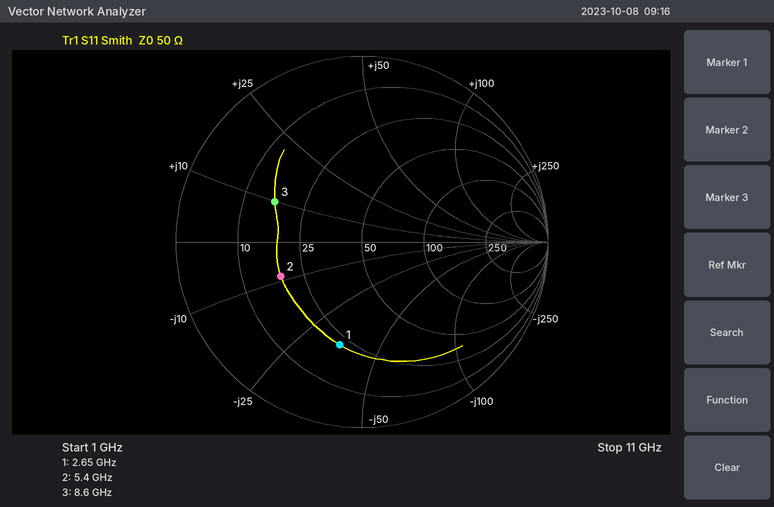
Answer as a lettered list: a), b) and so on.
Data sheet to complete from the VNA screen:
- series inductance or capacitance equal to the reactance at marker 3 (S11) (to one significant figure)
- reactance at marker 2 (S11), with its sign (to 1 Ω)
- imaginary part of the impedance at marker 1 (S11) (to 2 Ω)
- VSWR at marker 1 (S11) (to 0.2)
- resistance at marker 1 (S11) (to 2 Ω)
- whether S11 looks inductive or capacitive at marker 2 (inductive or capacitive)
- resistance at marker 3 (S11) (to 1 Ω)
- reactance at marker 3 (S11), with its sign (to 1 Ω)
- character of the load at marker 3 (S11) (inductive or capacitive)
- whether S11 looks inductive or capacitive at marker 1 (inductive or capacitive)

a) 200 pH
b) -9 Ω
c) -36 Ω
d) 3.6
e) 22 Ω
f) capacitive
g) 17 Ω
h) +10 Ω
i) inductive
j) capacitive
